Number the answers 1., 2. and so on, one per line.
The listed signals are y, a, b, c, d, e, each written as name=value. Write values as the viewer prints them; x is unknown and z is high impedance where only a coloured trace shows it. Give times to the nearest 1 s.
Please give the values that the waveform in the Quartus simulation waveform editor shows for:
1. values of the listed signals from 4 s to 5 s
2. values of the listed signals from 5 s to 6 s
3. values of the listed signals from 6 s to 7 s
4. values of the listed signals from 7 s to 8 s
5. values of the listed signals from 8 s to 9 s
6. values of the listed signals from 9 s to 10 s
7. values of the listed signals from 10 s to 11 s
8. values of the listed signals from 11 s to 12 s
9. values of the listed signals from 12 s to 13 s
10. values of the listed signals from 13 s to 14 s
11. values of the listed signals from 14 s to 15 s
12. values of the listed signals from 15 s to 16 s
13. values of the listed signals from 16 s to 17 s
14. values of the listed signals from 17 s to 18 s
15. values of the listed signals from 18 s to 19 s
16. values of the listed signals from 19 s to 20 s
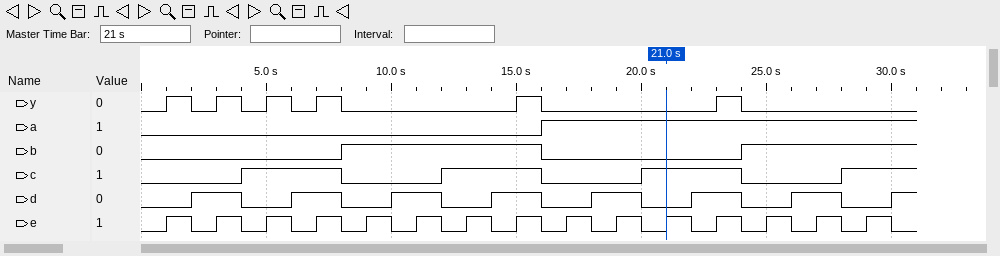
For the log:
1. y=0, a=0, b=0, c=1, d=0, e=0
2. y=1, a=0, b=0, c=1, d=0, e=1
3. y=0, a=0, b=0, c=1, d=1, e=0
4. y=1, a=0, b=0, c=1, d=1, e=1
5. y=0, a=0, b=1, c=0, d=0, e=0
6. y=0, a=0, b=1, c=0, d=0, e=1
7. y=0, a=0, b=1, c=0, d=1, e=0
8. y=0, a=0, b=1, c=0, d=1, e=1
9. y=0, a=0, b=1, c=1, d=0, e=0
10. y=0, a=0, b=1, c=1, d=0, e=1
11. y=0, a=0, b=1, c=1, d=1, e=0
12. y=1, a=0, b=1, c=1, d=1, e=1
13. y=0, a=1, b=0, c=0, d=0, e=0
14. y=0, a=1, b=0, c=0, d=0, e=1
15. y=0, a=1, b=0, c=0, d=1, e=0
16. y=0, a=1, b=0, c=0, d=1, e=1
